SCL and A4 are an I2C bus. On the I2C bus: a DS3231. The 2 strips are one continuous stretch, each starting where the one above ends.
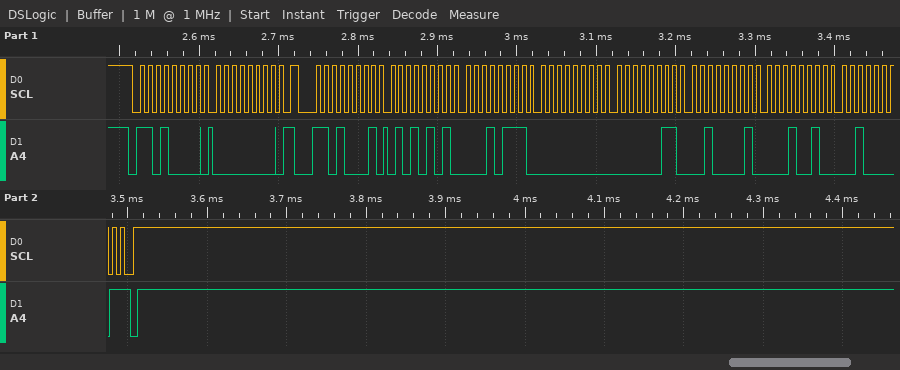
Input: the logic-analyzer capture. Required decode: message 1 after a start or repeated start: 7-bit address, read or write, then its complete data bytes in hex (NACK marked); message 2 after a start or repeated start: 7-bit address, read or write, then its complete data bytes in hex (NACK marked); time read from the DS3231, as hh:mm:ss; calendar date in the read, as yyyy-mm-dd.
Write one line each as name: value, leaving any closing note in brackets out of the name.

message 1 after a start or repeated start: 7-bit address, read or write, then its complete data bytes in hex: 0x68 write: 00
message 2 after a start or repeated start: 7-bit address, read or write, then its complete data bytes in hex: 0x68 read: 55 17 00 03 21 12 21 NACK
time read from the DS3231, as hh:mm:ss: 00:17:55
calendar date in the read, as yyyy-mm-dd: 2021-12-21
